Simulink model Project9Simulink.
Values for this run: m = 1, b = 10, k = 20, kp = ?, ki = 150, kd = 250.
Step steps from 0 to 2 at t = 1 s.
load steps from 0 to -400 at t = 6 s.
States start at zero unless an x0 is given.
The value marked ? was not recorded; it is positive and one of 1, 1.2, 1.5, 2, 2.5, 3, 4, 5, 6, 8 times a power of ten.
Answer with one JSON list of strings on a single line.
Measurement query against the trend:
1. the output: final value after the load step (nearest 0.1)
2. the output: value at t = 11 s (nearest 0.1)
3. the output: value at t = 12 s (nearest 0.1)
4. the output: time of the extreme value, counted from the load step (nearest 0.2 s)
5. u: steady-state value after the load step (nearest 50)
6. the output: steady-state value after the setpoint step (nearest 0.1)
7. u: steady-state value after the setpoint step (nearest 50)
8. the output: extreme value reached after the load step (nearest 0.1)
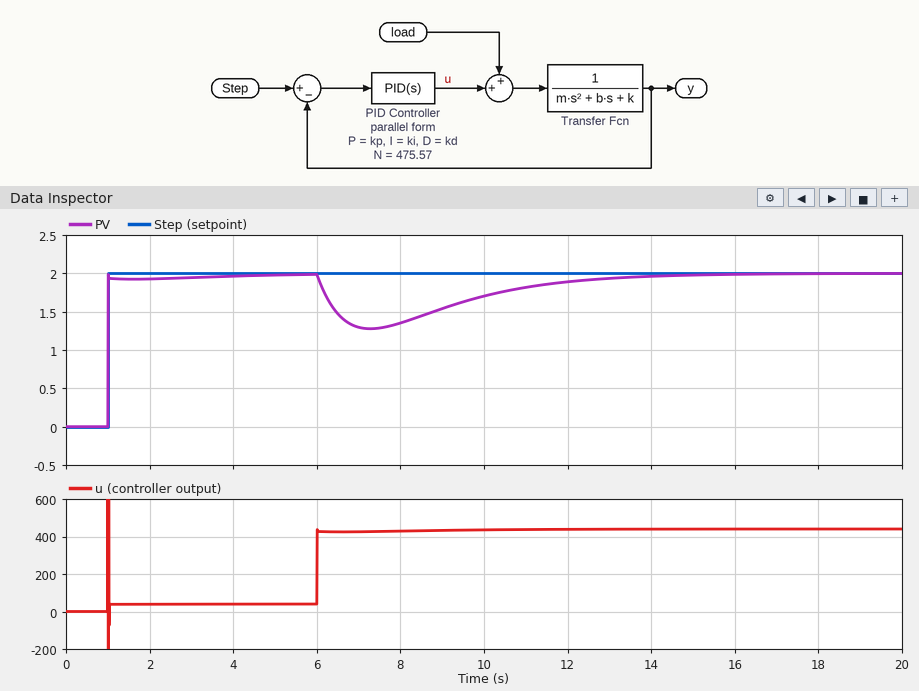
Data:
["2.0", "1.8", "1.9", "1.2 s", "450", "2.0", "50", "1.3"]
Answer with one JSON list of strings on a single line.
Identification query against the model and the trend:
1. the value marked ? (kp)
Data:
["400"]
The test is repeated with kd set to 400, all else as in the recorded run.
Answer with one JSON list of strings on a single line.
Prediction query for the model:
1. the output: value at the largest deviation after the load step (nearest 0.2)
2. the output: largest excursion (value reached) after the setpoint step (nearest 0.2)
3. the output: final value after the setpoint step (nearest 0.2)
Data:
["1.4", "2.2", "2.0"]
